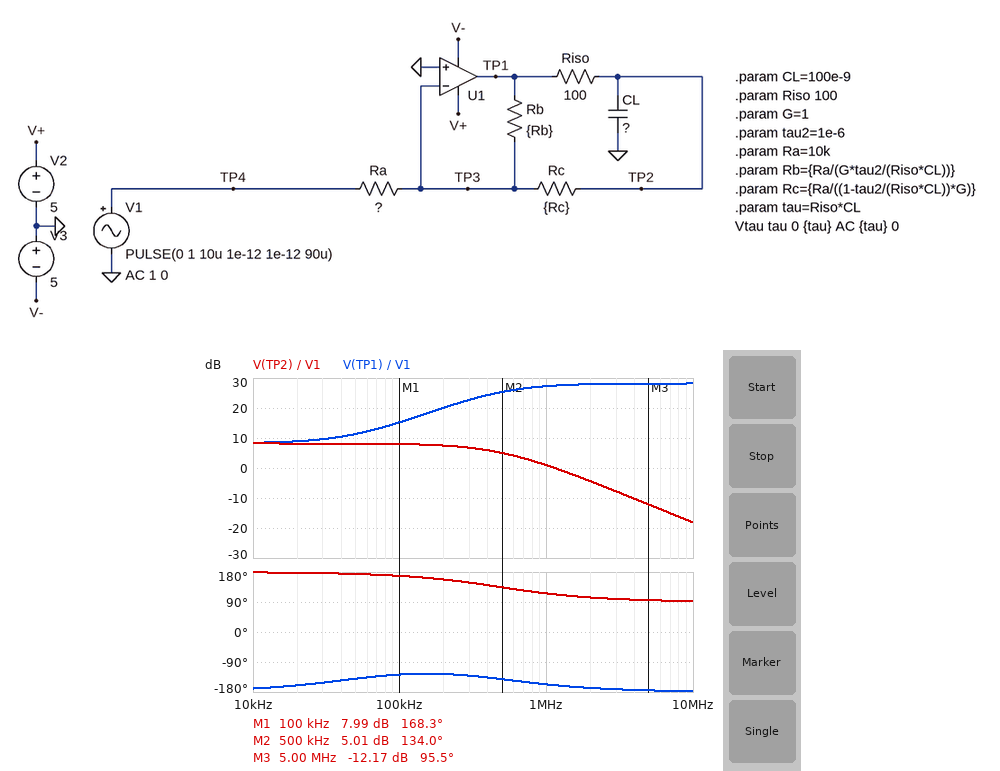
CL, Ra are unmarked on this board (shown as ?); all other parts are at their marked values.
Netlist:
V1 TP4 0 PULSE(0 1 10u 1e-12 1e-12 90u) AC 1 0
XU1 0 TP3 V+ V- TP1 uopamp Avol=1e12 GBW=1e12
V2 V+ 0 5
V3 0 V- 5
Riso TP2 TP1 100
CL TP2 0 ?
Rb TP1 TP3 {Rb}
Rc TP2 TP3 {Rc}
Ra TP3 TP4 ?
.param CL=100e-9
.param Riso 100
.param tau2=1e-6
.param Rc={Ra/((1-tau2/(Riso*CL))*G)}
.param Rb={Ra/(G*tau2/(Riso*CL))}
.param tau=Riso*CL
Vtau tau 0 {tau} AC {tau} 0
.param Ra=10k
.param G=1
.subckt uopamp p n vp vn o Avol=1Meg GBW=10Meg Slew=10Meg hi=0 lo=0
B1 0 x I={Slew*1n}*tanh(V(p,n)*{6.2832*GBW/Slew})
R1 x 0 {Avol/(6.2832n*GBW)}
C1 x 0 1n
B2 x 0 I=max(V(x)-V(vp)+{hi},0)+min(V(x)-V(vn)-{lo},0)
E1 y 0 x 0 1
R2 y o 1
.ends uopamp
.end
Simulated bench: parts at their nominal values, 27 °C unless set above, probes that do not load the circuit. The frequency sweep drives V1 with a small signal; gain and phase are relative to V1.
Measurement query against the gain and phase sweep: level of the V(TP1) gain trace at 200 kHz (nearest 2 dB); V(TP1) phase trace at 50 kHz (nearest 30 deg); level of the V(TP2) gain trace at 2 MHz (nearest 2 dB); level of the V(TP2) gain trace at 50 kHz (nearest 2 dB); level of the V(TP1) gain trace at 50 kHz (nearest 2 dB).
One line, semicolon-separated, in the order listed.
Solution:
20 dB; -150 deg; -4 dB; 8 dB; 12 dB
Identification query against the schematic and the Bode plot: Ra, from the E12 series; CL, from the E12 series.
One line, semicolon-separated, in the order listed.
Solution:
3.9 kΩ; 33 nF
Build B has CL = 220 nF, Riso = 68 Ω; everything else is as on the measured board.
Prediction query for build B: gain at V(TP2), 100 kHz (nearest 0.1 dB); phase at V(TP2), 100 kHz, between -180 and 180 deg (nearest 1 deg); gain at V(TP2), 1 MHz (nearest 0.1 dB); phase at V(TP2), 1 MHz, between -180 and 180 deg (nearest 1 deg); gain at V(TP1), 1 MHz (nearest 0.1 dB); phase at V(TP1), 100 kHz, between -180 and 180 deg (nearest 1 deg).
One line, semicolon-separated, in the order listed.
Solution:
5.4 dB; 137 deg; -11.3 dB; 96 deg; 28.1 dB; -139 deg
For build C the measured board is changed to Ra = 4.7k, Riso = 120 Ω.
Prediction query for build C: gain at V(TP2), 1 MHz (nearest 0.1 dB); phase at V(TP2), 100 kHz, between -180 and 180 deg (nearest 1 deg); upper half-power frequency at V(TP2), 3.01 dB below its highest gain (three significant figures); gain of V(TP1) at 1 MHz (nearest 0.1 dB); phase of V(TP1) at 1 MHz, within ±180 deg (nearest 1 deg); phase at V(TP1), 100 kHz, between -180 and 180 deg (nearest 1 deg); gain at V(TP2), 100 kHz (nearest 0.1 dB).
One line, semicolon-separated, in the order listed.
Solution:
-2.0 dB; 166 deg; 402 kHz; 25.9 dB; -160 deg; -126 deg; 6.3 dB
